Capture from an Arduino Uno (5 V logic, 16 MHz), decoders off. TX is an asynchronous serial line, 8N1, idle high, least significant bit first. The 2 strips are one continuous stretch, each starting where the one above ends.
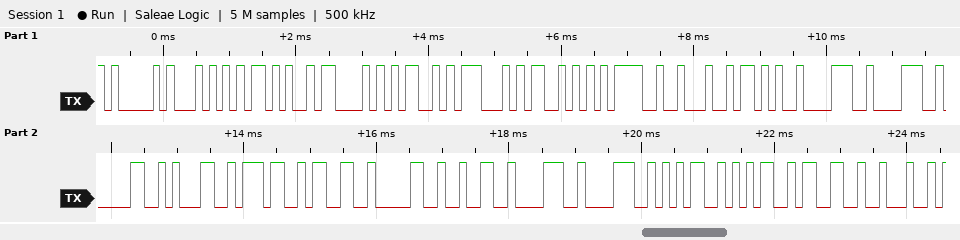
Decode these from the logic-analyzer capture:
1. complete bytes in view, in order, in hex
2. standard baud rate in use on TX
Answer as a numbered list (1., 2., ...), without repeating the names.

1. 41 54 2B 43 4D 47 53 3D 22 2B 38 38 30 31 37 33 30 32 38 38 35 35 33 22
2. 9600 baud
